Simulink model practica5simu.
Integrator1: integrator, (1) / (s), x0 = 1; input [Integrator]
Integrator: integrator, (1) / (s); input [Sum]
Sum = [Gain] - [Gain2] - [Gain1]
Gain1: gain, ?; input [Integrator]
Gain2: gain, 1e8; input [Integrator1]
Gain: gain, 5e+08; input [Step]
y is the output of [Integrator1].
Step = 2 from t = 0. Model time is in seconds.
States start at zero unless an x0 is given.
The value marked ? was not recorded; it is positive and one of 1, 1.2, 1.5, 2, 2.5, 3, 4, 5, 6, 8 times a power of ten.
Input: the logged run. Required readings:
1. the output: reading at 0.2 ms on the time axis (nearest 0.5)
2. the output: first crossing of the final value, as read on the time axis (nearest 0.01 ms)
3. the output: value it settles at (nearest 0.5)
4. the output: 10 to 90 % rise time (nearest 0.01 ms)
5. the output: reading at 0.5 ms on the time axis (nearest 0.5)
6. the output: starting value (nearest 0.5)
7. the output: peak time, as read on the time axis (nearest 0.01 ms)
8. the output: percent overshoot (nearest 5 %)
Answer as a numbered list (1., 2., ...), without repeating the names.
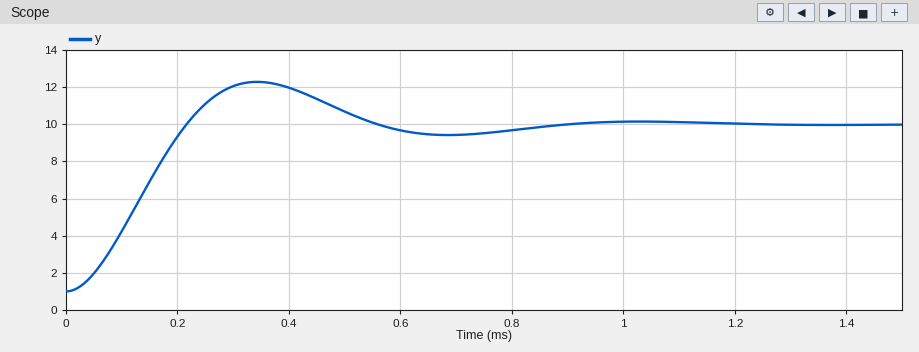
1. 9.5
2. 0.22 ms
3. 10.0
4. 0.15 ms
5. 10.5
6. 1.0
7. 0.34 ms
8. 25 %
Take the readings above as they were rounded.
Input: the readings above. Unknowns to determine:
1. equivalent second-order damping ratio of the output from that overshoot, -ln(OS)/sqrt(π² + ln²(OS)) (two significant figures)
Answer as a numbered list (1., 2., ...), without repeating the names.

1. 0.40
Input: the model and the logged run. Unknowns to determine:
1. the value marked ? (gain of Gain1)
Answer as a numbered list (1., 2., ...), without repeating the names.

1. 8000
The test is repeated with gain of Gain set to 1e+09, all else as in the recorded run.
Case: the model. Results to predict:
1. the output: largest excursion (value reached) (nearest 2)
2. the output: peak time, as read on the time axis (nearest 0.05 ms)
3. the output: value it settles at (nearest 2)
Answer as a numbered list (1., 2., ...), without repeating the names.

1. 24
2. 0.35 ms
3. 20
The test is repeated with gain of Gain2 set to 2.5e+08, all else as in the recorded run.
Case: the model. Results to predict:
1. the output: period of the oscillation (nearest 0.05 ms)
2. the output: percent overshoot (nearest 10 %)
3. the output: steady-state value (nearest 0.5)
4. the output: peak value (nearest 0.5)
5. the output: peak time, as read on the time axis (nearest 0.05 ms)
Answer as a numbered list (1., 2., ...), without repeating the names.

1. 0.40 ms
2. 40 %
3. 4.0
4. 5.5
5. 0.20 ms
